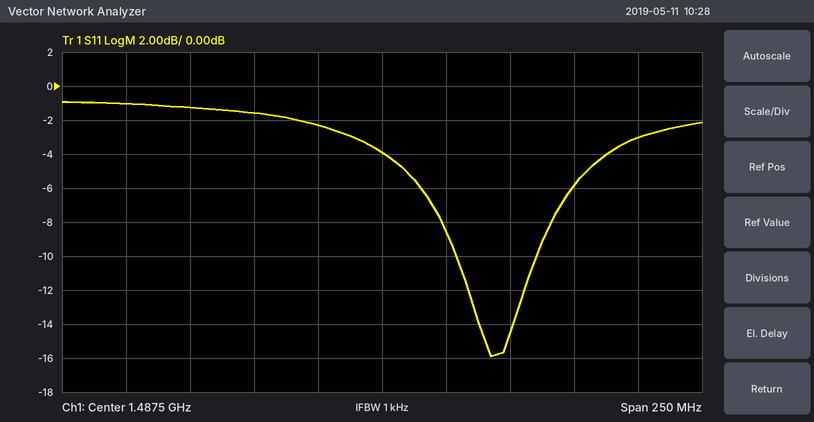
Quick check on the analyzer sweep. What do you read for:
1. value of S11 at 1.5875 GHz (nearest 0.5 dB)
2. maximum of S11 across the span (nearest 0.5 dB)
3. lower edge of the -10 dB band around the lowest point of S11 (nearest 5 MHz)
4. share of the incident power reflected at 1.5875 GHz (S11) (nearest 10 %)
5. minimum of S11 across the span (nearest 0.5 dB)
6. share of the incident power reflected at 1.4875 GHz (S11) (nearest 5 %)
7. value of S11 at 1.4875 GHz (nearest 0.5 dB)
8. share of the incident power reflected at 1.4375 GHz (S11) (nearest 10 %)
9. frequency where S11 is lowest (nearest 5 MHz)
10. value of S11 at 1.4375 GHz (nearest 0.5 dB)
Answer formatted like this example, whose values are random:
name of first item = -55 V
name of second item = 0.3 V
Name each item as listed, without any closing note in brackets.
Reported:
value of S11 at 1.5875 GHz = -3.0 dB
maximum of S11 across the span = -1.0 dB
lower edge of the -10 dB band around the lowest point of S11 = 1.515 GHz
share of the incident power reflected at 1.5875 GHz (S11) = 50 %
minimum of S11 across the span = -16.0 dB
share of the incident power reflected at 1.4875 GHz (S11) = 40 %
value of S11 at 1.4875 GHz = -4.0 dB
share of the incident power reflected at 1.4375 GHz (S11) = 70 %
frequency where S11 is lowest = 1.530 GHz
value of S11 at 1.4375 GHz = -1.5 dB
